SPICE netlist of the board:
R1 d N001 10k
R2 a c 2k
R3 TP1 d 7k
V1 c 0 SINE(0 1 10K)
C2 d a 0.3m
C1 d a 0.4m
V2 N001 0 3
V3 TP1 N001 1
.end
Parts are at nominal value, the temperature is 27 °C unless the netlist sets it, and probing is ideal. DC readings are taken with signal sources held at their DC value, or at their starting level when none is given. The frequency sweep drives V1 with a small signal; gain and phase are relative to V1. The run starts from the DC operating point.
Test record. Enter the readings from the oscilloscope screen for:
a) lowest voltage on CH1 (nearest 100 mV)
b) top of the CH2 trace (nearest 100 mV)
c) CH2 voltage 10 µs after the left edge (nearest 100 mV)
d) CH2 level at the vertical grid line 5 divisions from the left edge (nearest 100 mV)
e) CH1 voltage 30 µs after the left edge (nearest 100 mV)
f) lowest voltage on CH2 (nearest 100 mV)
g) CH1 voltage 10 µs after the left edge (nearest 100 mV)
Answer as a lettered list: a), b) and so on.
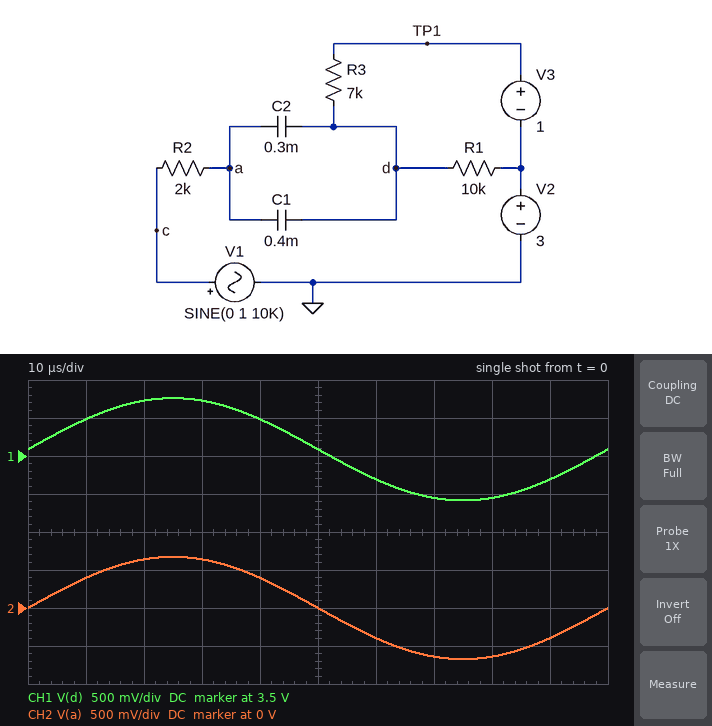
a) 2.9 V
b) 700 mV
c) 400 mV
d) 0 V
e) 4.2 V
f) -700 mV
g) 4.0 V
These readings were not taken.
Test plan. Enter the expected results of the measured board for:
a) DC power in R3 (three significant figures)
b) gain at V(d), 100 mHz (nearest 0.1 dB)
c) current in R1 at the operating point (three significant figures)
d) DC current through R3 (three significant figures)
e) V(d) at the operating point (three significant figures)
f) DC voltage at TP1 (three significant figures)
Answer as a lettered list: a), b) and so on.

a) 24.2 µW
b) -4.0 dB
c) 58.8 µA
d) 58.8 µA
e) 3.59 V
f) 4.00 V
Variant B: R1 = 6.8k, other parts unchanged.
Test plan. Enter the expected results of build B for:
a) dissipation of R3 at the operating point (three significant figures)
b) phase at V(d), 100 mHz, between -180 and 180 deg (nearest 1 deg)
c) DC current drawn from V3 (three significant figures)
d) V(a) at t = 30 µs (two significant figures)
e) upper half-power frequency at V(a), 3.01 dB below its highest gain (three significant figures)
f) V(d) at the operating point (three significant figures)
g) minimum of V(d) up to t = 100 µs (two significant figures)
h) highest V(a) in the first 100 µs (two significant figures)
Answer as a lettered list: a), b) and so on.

a) 36.8 µW
b) 23 deg
c) 72.5 µA
d) 600 mV
e) 93.6 mHz
f) 3.49 V
g) 2.9 V
h) 630 mV
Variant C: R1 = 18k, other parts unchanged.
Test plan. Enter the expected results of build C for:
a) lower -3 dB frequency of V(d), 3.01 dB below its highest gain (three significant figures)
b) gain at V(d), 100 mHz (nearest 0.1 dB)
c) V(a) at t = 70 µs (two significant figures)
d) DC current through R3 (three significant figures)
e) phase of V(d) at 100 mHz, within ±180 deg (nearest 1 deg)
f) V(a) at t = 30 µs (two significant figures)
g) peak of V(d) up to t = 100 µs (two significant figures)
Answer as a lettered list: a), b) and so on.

a) 32.3 mHz
b) -3.3 dB
c) -680 mV
d) 40.0 µA
e) 18 deg
f) 680 mV
g) 4.4 V
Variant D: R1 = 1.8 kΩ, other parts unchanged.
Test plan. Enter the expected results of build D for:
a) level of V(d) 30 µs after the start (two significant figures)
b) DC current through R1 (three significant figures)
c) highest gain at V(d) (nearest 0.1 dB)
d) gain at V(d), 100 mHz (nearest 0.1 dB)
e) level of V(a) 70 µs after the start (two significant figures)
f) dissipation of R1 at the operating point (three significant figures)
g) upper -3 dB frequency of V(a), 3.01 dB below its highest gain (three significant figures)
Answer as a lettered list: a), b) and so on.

a) 3.6 V
b) 114 µA
c) -7.6 dB
d) -9.2 dB
e) -400 mV
f) 23.2 µW
g) 82.1 mHz
